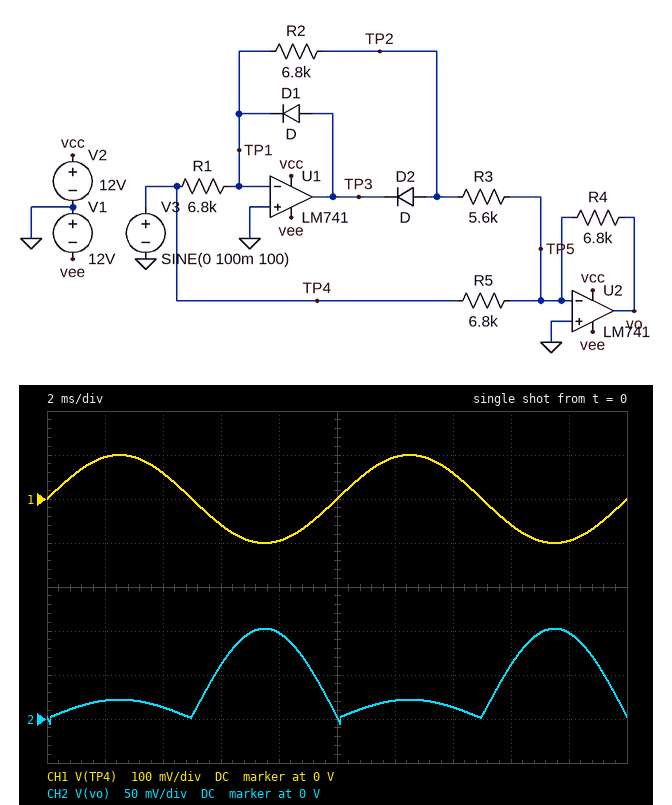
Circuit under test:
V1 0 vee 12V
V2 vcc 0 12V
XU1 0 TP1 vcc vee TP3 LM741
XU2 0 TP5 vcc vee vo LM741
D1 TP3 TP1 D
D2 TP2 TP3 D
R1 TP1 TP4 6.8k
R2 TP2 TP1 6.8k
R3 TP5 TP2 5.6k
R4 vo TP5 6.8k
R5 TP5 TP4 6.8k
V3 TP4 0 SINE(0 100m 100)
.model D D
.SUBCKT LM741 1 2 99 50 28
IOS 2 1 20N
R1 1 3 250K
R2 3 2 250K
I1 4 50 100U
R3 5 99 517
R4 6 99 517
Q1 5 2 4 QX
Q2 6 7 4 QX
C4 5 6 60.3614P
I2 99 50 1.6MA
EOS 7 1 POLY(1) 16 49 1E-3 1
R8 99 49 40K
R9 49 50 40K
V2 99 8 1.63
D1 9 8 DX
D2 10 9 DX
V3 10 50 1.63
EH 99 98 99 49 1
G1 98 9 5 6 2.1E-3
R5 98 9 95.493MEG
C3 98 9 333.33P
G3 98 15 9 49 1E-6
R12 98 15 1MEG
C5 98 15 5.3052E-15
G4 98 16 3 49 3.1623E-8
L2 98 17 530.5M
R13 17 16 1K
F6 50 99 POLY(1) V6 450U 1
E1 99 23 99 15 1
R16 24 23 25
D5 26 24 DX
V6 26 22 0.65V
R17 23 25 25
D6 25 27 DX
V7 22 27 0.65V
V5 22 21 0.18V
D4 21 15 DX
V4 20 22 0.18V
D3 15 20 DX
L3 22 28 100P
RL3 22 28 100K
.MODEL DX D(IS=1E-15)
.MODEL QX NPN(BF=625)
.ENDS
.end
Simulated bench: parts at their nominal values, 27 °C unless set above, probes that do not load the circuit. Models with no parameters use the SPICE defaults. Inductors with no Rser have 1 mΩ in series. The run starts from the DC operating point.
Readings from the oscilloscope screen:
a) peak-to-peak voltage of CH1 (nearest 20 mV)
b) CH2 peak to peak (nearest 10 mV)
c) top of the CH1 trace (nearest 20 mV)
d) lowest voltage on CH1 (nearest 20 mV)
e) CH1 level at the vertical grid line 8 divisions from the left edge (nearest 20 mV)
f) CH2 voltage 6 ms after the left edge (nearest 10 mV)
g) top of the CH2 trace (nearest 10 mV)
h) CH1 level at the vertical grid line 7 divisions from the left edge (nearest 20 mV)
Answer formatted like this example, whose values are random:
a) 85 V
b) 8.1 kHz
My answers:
a) 200 mV
b) 110 mV
c) 100 mV
d) -100 mV
e) -60 mV
f) 60 mV
g) 100 mV
h) 60 mV
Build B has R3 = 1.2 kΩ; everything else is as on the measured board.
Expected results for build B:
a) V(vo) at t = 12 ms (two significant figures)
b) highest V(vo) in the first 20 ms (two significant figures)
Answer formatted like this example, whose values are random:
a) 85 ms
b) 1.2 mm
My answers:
a) 440 mV
b) 460 mV
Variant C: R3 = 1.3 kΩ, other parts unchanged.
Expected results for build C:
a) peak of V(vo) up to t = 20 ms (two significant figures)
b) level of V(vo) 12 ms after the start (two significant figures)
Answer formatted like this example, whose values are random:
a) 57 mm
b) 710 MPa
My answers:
a) 420 mV
b) 400 mV
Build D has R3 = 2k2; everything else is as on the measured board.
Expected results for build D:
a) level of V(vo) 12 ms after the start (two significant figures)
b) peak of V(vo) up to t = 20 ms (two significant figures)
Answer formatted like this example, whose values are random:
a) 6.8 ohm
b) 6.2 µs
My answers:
a) 200 mV
b) 210 mV
